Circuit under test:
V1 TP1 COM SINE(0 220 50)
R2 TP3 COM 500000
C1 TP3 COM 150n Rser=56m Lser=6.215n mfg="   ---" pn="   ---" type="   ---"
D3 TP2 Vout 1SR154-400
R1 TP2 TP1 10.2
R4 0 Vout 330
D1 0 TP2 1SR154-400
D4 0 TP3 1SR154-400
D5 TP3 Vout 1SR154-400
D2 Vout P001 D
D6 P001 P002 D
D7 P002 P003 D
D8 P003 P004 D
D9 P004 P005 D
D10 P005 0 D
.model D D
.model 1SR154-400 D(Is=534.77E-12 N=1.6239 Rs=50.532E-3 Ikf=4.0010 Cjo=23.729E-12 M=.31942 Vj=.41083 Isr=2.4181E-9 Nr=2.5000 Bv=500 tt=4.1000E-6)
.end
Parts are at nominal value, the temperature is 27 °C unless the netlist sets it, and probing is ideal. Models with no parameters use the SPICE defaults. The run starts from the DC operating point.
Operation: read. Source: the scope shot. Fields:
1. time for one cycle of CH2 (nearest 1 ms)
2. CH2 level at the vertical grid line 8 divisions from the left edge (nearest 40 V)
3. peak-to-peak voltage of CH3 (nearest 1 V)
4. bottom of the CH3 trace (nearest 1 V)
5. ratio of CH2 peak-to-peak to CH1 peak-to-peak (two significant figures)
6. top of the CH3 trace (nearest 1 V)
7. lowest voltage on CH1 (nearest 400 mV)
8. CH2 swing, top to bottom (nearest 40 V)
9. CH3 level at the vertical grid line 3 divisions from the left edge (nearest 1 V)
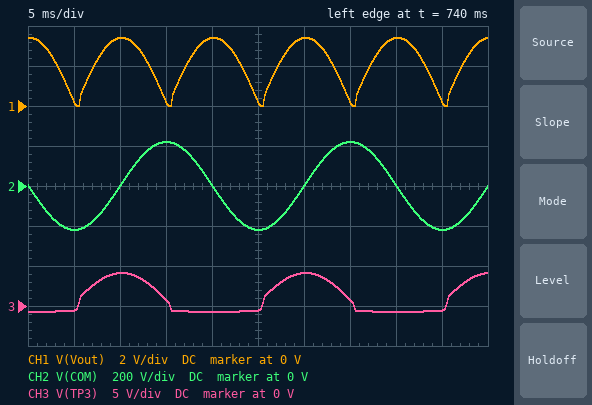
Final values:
20 ms
0 V
5 V
-1 V
130
4 V
0 V
440 V
1 V
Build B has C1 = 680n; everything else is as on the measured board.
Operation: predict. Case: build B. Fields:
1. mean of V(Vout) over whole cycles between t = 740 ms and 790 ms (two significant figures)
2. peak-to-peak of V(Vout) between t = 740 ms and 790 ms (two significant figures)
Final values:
3.9 V
4.5 V
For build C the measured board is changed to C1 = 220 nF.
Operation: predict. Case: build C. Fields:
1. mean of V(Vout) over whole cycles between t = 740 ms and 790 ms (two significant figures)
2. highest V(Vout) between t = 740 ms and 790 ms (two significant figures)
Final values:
2.9 V
4.1 V
